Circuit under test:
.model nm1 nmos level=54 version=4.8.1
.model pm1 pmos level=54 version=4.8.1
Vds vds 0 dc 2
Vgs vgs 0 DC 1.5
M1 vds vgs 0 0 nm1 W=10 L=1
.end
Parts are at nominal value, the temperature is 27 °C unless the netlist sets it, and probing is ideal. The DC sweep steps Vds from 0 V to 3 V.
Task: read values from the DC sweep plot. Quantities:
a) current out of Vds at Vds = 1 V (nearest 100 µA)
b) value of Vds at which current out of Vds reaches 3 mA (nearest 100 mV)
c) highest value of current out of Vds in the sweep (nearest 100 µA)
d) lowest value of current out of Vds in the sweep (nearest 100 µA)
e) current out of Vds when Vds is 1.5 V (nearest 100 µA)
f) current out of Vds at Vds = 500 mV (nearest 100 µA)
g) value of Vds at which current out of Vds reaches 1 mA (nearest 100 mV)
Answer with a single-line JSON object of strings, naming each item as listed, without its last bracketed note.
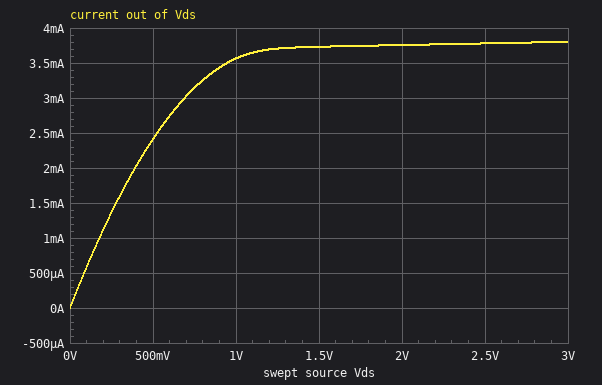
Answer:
{"current out of Vds at Vds = 1 V": "3.6 mA", "value of Vds at which current out of Vds reaches 3 mA": "700 mV", "highest value of current out of Vds in the sweep": "3.8 mA", "lowest value of current out of Vds in the sweep": "0 A", "current out of Vds when Vds is 1.5 V": "3.7 mA", "current out of Vds at Vds = 500 mV": "2.4 mA", "value of Vds at which current out of Vds reaches 1 mA": "200 mV"}
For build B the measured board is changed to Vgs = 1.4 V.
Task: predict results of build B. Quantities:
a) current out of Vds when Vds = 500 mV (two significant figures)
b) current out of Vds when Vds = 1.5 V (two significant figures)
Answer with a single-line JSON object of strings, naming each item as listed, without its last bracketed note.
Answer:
{"current out of Vds when Vds = 500 mV": "2.2 mA", "current out of Vds when Vds = 1.5 V": "3.3 mA"}
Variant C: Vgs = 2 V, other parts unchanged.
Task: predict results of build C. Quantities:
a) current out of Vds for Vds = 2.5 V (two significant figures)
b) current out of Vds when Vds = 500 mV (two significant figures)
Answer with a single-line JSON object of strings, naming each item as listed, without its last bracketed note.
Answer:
{"current out of Vds for Vds = 2.5 V": "6.3 mA", "current out of Vds when Vds = 500 mV": "3.2 mA"}
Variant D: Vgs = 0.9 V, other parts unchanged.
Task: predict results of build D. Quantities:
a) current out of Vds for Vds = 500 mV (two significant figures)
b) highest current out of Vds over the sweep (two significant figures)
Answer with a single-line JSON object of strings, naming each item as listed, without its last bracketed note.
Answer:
{"current out of Vds for Vds = 500 mV": "1.2 mA", "highest current out of Vds over the sweep": "1.4 mA"}
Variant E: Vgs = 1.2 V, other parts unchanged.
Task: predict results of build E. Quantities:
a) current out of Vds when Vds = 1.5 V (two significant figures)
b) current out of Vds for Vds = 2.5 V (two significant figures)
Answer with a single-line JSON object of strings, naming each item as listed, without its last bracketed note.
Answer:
{"current out of Vds when Vds = 1.5 V": "2.4 mA", "current out of Vds for Vds = 2.5 V": "2.5 mA"}
